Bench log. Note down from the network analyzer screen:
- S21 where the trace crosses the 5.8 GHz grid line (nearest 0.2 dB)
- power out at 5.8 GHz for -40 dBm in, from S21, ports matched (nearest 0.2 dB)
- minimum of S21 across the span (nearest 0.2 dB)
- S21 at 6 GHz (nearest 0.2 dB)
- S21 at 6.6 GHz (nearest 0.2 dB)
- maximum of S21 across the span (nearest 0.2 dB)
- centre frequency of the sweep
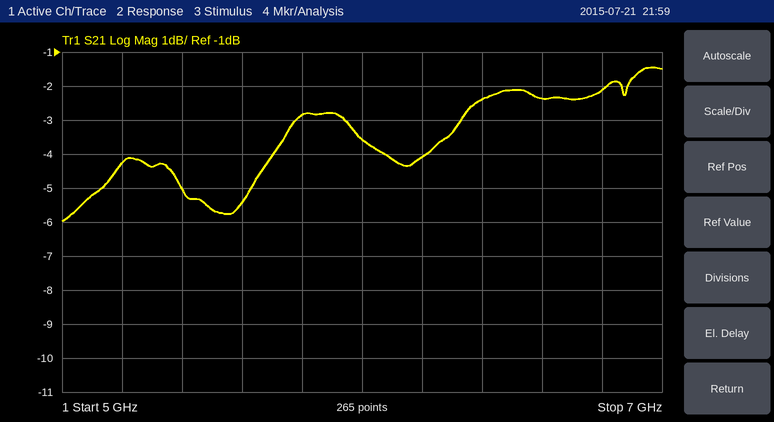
-2.8 dB
-42.8 dBm
-6.0 dB
-3.6 dB
-2.4 dB
-1.4 dB
6 GHz
